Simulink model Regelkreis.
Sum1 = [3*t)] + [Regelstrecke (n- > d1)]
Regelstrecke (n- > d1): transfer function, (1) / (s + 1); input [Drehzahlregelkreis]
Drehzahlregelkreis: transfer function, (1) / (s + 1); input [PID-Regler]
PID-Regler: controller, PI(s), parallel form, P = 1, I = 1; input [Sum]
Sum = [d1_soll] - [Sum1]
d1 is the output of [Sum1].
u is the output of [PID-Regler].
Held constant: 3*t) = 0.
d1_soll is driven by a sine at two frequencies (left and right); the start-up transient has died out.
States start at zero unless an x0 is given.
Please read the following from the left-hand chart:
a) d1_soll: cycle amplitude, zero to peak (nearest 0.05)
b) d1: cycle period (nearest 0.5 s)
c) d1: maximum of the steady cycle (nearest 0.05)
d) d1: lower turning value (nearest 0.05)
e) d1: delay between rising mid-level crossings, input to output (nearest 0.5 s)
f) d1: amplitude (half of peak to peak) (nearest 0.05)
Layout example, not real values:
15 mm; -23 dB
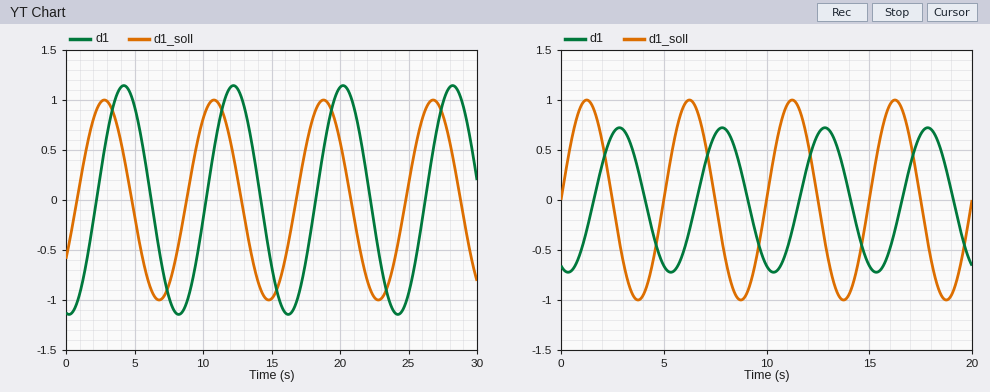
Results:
1.00; 8.0 s; 1.15; -1.15; 1.5 s; 1.15
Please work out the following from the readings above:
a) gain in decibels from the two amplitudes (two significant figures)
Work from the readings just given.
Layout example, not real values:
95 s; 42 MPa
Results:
1.2 dB
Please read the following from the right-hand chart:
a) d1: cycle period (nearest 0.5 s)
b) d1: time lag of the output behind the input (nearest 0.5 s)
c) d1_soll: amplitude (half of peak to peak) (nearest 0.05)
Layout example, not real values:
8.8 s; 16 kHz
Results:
5.0 s; 1.5 s; 1.00
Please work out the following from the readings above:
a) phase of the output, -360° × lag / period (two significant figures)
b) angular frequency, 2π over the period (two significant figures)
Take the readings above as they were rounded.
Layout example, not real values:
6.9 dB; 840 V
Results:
-110°; 1.3 rad/s
